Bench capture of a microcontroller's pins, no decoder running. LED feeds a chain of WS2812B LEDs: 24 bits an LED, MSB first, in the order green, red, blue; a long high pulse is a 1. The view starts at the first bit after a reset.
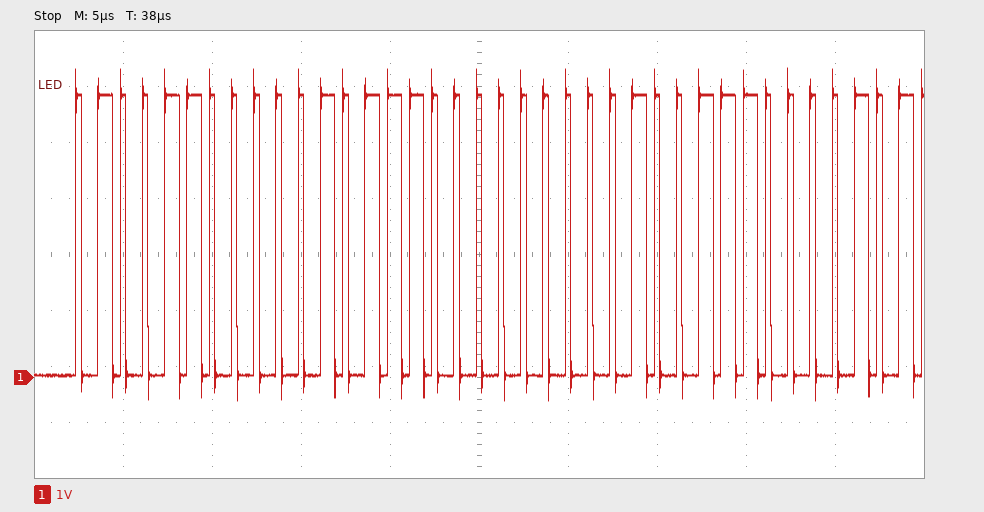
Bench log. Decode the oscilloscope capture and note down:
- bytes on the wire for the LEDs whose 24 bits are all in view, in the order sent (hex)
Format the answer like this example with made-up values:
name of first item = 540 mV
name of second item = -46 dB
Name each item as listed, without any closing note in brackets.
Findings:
bytes on the wire for the LEDs whose 24 bits are all in view, in the order sent = 4C 17 00
